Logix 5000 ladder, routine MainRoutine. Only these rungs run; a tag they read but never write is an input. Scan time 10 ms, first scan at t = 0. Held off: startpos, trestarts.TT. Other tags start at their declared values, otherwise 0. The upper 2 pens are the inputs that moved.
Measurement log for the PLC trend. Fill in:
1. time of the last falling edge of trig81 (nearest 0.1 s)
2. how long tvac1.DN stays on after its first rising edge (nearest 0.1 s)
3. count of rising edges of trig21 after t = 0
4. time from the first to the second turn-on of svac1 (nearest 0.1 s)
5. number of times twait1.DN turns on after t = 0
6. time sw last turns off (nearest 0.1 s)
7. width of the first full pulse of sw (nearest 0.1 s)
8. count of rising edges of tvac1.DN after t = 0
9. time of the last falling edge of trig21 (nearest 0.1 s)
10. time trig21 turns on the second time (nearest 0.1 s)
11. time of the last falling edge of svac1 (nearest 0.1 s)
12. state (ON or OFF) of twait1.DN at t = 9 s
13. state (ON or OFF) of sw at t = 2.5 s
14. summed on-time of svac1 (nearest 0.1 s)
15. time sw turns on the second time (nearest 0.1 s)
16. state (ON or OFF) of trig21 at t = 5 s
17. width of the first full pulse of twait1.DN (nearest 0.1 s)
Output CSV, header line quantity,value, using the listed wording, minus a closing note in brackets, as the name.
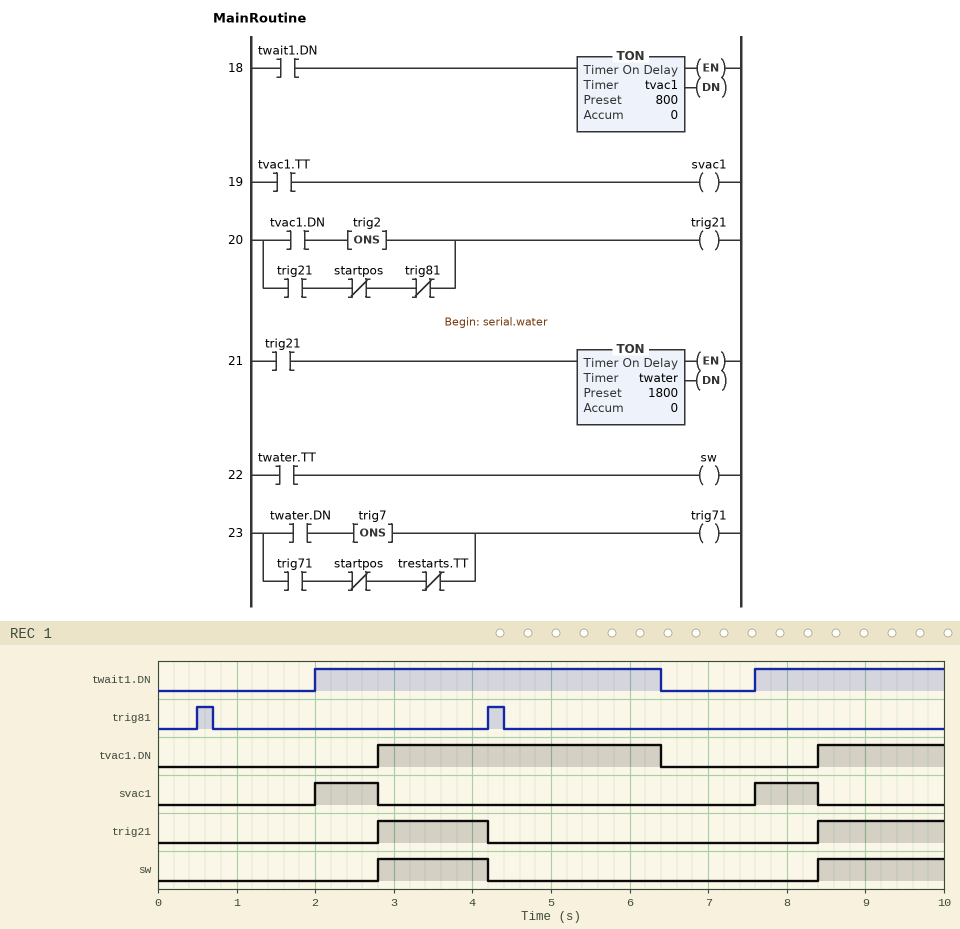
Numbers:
quantity,value
time of the last falling edge of trig81,4.4 s
how long tvac1.DN stays on after its first rising edge,3.6 s
count of rising edges of trig21 after t = 0,2
time from the first to the second turn-on of svac1,5.6 s
number of times twait1.DN turns on after t = 0,2
time sw last turns off,4.2 s
width of the first full pulse of sw,1.4 s
count of rising edges of tvac1.DN after t = 0,2
time of the last falling edge of trig21,4.2 s
time trig21 turns on the second time,8.4 s
time of the last falling edge of svac1,8.4 s
state (ON or OFF) of twait1.DN at t = 9 s,ON
state (ON or OFF) of sw at t = 2.5 s,OFF
summed on-time of svac1,1.6 s
time sw turns on the second time,8.4 s
state (ON or OFF) of trig21 at t = 5 s,OFF
width of the first full pulse of twait1.DN,4.4 s
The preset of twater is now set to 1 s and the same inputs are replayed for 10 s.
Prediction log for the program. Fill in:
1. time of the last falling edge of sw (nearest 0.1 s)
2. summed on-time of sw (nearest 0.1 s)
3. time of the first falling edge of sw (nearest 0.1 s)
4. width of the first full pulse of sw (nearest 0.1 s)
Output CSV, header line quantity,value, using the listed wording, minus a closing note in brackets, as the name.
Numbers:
quantity,value
time of the last falling edge of sw,9.4 s
summed on-time of sw,2.0 s
time of the first falling edge of sw,3.8 s
width of the first full pulse of sw,1.0 s
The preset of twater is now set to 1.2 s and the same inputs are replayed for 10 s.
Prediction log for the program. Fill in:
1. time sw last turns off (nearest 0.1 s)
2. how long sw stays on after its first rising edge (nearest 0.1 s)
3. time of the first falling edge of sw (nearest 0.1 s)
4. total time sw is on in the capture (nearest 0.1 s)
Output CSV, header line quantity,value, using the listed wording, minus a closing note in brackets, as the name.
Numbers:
quantity,value
time sw last turns off,9.6 s
how long sw stays on after its first rising edge,1.2 s
time of the first falling edge of sw,4.0 s
total time sw is on in the capture,2.4 s
